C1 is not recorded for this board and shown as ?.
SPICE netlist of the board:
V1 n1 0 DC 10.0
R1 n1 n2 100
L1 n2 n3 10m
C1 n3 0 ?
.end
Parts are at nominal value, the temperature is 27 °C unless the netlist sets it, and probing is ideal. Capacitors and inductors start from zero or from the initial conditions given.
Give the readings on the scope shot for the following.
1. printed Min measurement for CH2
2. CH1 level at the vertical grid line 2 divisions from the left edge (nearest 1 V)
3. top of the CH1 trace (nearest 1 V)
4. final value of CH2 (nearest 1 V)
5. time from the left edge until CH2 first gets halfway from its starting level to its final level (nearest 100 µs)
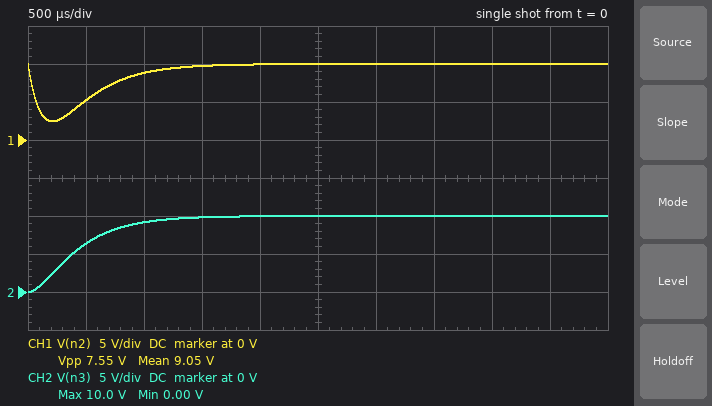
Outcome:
0.00 V
9 V
10 V
10 V
400 µs
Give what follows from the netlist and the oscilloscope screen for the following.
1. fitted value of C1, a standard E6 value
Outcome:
4.7 µF
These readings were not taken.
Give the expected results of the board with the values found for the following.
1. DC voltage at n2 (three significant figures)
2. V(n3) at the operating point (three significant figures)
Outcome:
10.0 V
10.0 V
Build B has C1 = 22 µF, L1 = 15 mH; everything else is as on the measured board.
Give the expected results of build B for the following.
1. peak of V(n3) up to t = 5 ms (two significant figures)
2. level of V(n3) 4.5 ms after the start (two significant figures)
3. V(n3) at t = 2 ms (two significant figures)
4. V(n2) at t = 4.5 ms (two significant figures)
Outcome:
9.1 V
8.8 V
5.9 V
8.7 V
